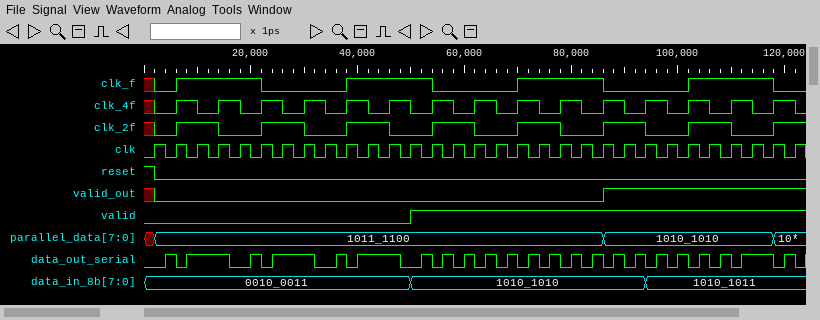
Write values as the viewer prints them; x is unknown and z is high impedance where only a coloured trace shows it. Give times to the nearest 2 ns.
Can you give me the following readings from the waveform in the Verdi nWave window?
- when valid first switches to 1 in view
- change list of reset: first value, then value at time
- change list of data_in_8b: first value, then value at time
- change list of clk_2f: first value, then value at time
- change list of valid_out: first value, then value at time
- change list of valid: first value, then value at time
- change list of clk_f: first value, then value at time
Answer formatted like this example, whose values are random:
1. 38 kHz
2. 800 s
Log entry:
1. 50 ns
2. 1, 0 at 2 ns
3. 0010_0011, 1010_1010 at 50 ns, 1010_1011 at 94 ns
4. x, 0 at 2 ns, 1 at 6 ns, 0 at 14 ns, 1 at 22 ns, 0 at 30 ns, 1 at 38 ns, 0 at 46 ns, 1 at 54 ns, 0 at 62 ns, 1 at 70 ns, 0 at 78 ns, 1 at 86 ns, 0 at 94 ns, 1 at 102 ns, 0 at 110 ns, 1 at 118 ns
5. x, 0 at 2 ns, 1 at 86 ns
6. 0, 1 at 50 ns
7. x, 0 at 2 ns, 1 at 6 ns, 0 at 22 ns, 1 at 38 ns, 0 at 54 ns, 1 at 70 ns, 0 at 86 ns, 1 at 102 ns, 0 at 118 ns
